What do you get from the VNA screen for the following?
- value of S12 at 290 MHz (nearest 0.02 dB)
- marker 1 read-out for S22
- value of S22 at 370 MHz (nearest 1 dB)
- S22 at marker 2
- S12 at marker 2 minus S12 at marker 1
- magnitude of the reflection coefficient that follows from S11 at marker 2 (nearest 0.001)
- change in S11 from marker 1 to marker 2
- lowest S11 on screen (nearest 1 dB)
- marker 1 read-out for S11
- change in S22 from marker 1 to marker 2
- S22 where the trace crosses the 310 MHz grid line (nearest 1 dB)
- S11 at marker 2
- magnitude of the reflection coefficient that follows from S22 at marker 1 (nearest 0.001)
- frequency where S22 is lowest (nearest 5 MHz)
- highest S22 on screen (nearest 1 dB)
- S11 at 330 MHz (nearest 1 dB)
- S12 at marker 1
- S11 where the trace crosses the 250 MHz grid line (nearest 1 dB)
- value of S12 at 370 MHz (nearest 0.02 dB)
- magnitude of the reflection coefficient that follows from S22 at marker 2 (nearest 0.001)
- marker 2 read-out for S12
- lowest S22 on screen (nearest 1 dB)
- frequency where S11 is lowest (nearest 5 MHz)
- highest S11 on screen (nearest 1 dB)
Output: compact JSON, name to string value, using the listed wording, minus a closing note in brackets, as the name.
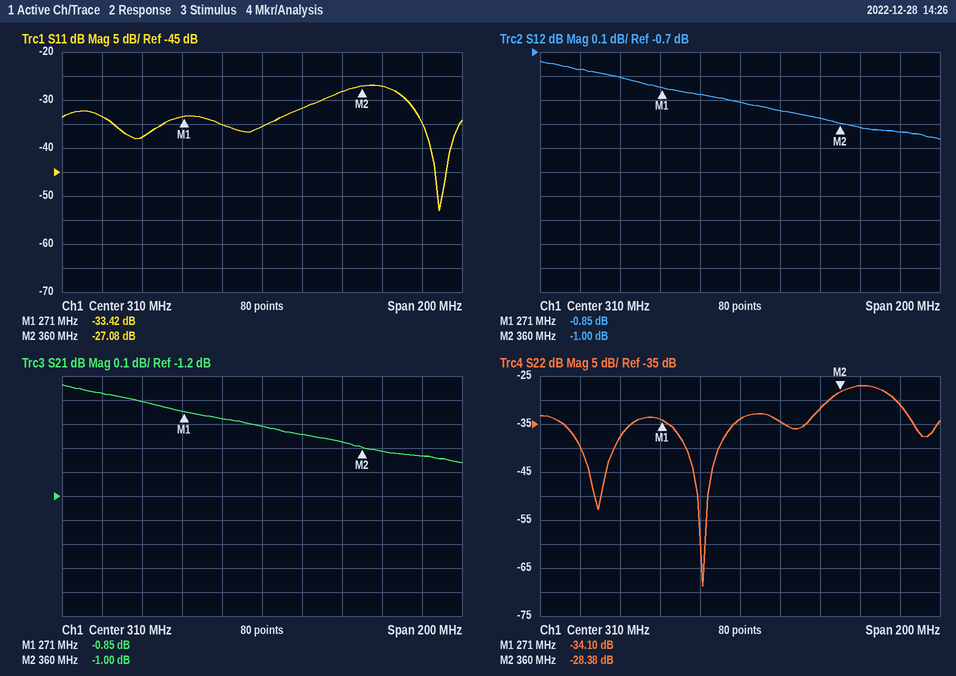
{"value of S12 at 290 MHz": "-0.88 dB", "marker 1 read-out for S22": "-34.10 dB", "value of S22 at 370 MHz": "-27 dB", "S22 at marker 2": "-28.38 dB", "S12 at marker 2 minus S12 at marker 1": "-0.15 dB", "magnitude of the reflection coefficient that follows from S11 at marker 2": "0.044", "change in S11 from marker 1 to marker 2": "6.34 dB", "lowest S11 on screen": "-53 dB", "marker 1 read-out for S11": "-33.42 dB", "change in S22 from marker 1 to marker 2": "5.72 dB", "S22 where the trace crosses the 310 MHz grid line": "-34 dB", "S11 at marker 2": "-27.08 dB", "magnitude of the reflection coefficient that follows from S22 at marker 1": "0.020", "frequency where S22 is lowest": "290 MHz", "highest S22 on screen": "-27 dB", "S11 at 330 MHz": "-32 dB", "S12 at marker 1": "-0.85 dB", "S11 where the trace crosses the 250 MHz grid line": "-38 dB", "value of S12 at 370 MHz": "-1.02 dB", "magnitude of the reflection coefficient that follows from S22 at marker 2": "0.038", "marker 2 read-out for S12": "-1.00 dB", "lowest S22 on screen": "-69 dB", "frequency where S11 is lowest": "400 MHz", "highest S11 on screen": "-27 dB"}
